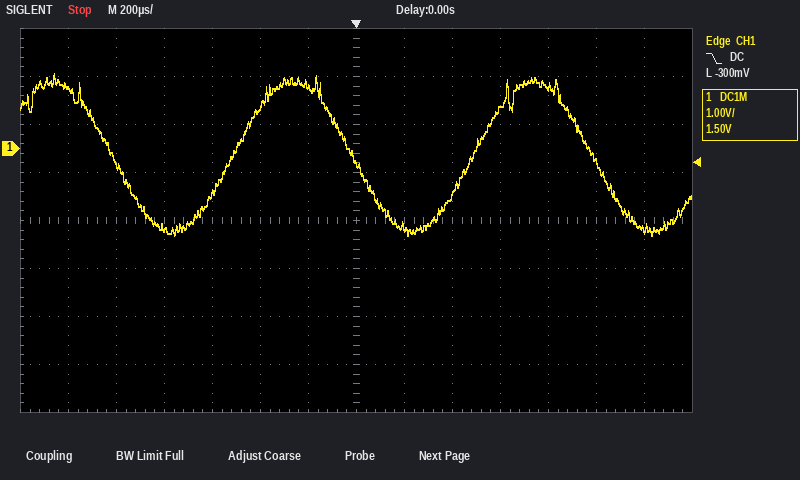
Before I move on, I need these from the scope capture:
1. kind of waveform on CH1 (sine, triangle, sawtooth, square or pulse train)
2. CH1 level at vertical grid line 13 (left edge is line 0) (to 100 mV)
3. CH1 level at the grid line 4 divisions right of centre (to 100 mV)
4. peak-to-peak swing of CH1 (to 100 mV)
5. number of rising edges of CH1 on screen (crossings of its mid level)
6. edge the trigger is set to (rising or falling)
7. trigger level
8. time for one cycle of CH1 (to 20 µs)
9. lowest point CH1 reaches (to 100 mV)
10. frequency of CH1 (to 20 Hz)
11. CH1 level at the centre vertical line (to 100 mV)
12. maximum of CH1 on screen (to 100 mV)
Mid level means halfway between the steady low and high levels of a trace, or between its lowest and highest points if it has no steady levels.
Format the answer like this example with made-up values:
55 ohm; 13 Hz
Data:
sine; -1.7 V; 1.3 V; 3.4 V; 2; falling; -300 mV; 1.00 ms; -1.8 V; 1.00 kHz; -300 mV; 1.6 V
